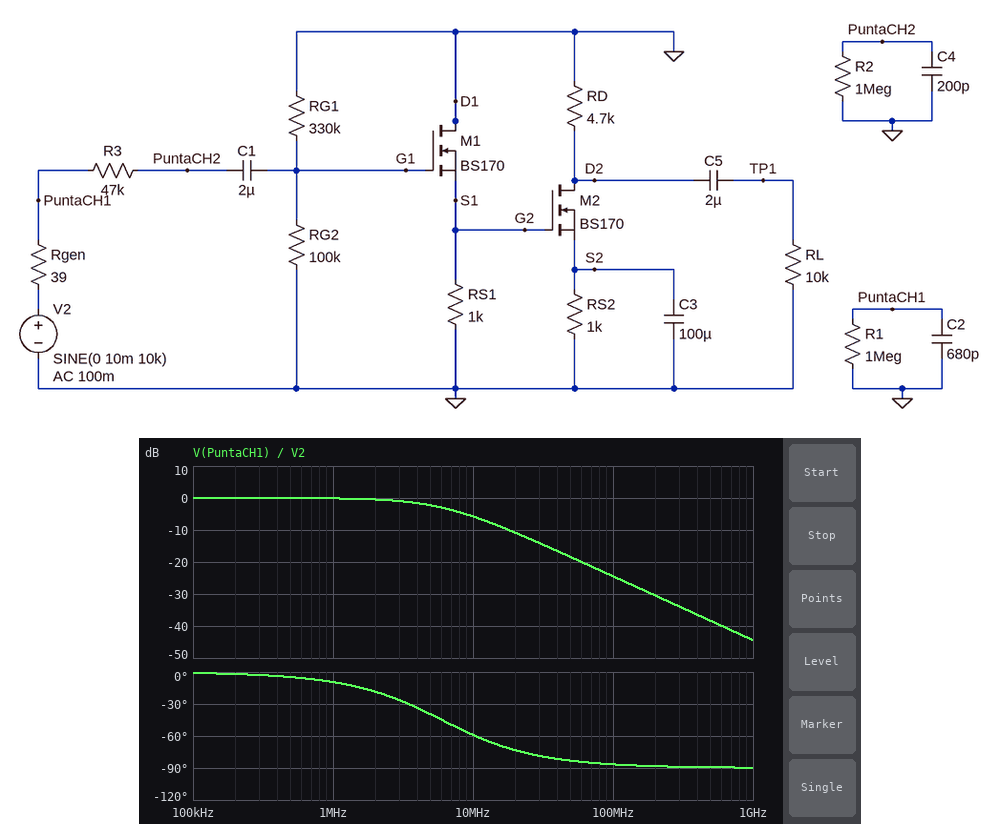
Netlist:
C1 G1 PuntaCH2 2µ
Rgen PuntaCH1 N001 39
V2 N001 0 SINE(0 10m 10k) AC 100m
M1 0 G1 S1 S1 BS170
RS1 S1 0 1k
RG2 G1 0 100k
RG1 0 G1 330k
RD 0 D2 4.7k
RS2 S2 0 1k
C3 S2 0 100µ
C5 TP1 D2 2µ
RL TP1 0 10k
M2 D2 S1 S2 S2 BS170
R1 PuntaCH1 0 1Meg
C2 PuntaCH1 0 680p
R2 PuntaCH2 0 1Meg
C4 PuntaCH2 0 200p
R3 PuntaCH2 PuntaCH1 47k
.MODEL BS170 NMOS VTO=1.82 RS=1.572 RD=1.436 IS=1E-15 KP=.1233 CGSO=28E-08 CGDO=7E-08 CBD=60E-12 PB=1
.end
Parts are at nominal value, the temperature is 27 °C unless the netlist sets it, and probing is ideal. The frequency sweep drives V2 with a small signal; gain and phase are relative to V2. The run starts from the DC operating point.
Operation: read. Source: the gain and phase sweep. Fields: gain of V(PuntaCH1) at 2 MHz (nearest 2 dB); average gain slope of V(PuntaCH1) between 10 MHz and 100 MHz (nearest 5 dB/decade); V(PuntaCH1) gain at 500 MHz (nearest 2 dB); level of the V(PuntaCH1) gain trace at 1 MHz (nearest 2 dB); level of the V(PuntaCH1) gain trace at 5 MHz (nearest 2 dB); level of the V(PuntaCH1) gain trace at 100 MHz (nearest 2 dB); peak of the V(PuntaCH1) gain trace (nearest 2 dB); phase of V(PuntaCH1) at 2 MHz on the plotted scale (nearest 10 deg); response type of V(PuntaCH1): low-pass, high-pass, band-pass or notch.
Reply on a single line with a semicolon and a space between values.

0 dB; -20 dB/decade; -38 dB; 0 dB; -2 dB; -24 dB; 0 dB; -20 deg; low-pass
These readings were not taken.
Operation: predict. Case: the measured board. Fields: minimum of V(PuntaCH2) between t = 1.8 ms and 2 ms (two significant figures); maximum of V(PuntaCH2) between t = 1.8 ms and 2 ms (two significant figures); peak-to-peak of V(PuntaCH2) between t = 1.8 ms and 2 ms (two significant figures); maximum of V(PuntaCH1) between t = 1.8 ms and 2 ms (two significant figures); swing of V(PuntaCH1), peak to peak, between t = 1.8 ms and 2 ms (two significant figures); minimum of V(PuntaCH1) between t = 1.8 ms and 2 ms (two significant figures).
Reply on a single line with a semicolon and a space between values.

-5.6 mV; 5.6 mV; 11 mV; 10 mV; 20 mV; -10 mV
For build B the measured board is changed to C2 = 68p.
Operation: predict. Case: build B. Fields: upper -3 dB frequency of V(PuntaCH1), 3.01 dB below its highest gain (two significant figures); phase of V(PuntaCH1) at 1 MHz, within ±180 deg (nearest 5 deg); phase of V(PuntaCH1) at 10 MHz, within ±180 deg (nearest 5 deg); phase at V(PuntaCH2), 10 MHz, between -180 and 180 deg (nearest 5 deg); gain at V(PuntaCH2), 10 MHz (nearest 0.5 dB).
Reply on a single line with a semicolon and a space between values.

60 MHz; 0 deg; -10 deg; -100 deg; -56.5 dB
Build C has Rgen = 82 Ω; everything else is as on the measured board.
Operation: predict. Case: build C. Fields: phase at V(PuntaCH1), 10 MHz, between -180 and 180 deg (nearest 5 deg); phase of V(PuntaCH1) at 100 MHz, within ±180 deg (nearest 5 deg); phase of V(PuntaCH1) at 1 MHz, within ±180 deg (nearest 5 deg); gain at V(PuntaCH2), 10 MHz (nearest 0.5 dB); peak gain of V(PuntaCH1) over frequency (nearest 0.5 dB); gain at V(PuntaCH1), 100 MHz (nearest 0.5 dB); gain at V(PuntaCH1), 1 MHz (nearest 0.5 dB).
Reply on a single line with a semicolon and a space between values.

-75 deg; -90 deg; -20 deg; -68.0 dB; 0 dB; -31.0 dB; -0.5 dB
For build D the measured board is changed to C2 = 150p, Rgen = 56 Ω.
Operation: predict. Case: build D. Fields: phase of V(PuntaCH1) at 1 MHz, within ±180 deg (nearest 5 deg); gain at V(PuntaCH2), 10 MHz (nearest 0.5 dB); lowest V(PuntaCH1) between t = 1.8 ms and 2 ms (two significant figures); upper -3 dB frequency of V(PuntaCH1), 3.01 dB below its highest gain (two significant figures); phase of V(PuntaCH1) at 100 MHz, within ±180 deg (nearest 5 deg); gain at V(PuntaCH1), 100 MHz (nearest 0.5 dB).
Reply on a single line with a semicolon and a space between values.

-5 deg; -57.5 dB; -10 mV; 19 MHz; -80 deg; -14.5 dB
